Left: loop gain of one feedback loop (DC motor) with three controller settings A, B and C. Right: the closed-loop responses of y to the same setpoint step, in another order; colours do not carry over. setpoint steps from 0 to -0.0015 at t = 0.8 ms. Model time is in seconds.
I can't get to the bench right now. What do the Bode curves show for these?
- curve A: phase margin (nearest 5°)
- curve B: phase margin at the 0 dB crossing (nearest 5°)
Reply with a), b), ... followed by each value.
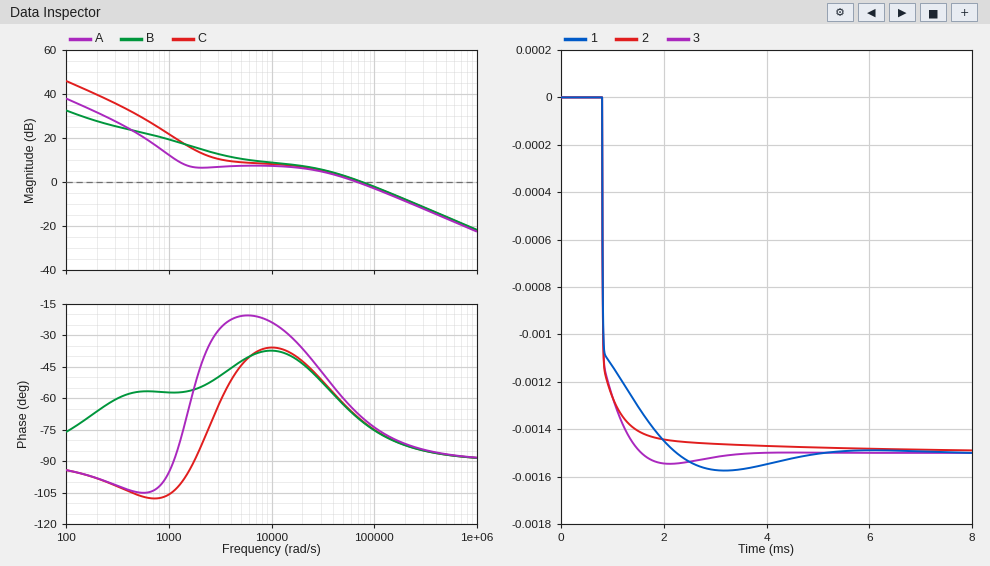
a) 115°
b) 110°
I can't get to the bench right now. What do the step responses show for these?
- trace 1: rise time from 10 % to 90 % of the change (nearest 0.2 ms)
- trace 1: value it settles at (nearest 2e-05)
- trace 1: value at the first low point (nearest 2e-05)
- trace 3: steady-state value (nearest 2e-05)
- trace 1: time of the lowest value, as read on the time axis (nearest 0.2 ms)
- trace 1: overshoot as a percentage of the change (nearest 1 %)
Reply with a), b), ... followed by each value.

a) 0.8 ms
b) -0.00150
c) -0.00158
d) -0.00150
e) 3.2 ms
f) 5 %
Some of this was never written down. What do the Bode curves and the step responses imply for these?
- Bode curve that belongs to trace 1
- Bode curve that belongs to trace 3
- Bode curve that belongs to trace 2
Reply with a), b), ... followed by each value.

a) A
b) C
c) B
